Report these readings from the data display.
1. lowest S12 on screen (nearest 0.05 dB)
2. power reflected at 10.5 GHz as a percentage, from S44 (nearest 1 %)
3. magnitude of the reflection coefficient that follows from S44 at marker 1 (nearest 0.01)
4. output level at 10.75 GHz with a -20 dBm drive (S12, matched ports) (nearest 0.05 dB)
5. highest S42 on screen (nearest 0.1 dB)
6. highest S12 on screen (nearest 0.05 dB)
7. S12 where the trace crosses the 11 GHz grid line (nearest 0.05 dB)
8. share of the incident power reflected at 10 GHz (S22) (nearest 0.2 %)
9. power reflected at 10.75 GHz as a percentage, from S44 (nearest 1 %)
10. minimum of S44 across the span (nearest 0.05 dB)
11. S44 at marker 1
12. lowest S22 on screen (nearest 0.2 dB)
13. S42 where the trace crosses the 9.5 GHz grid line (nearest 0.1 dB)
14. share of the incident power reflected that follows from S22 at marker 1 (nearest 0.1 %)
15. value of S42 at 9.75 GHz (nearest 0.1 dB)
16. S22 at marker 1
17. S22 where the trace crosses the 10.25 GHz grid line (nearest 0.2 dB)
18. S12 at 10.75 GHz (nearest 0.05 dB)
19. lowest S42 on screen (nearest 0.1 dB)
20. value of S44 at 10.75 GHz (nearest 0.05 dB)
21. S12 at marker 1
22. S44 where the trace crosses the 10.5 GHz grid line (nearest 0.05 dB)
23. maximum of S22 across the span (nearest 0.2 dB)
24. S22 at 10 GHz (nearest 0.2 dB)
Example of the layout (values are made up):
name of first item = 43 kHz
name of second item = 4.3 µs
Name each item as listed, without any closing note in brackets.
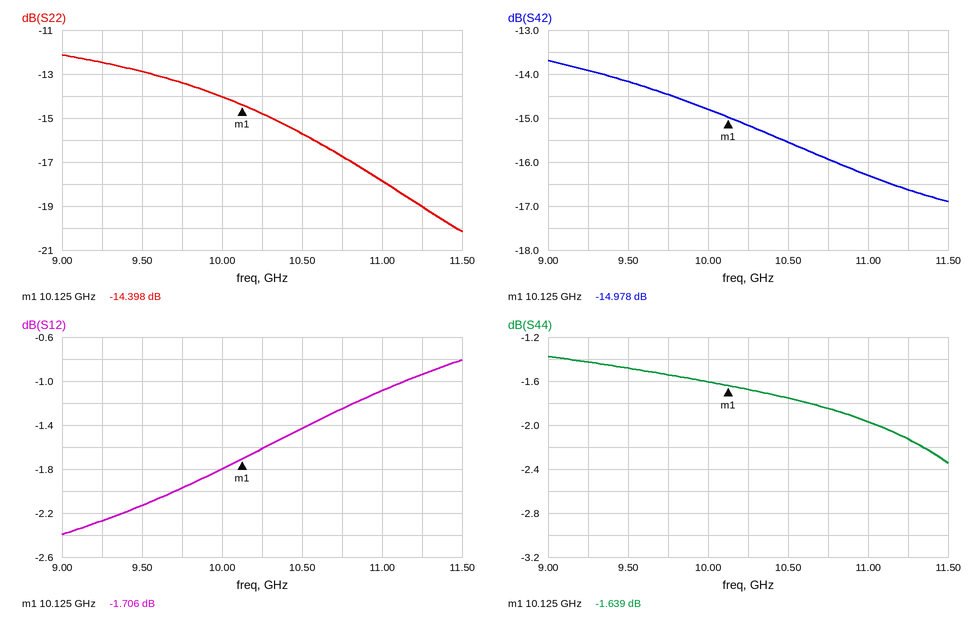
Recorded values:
lowest S12 on screen = -2.40 dB
power reflected at 10.5 GHz as a percentage, from S44 = 67 %
magnitude of the reflection coefficient that follows from S44 at marker 1 = 0.83
output level at 10.75 GHz with a -20 dBm drive (S12, matched ports) = -21.25 dBm
highest S42 on screen = -13.7 dB
highest S12 on screen = -0.80 dB
S12 where the trace crosses the 11 GHz grid line = -1.10 dB
share of the incident power reflected at 10 GHz (S22) = 4.0 %
power reflected at 10.75 GHz as a percentage, from S44 = 65 %
minimum of S44 across the span = -2.35 dB
S44 at marker 1 = -1.639 dB
lowest S22 on screen = -20.2 dB
S42 where the trace crosses the 9.5 GHz grid line = -14.2 dB
share of the incident power reflected that follows from S22 at marker 1 = 3.6 %
value of S42 at 9.75 GHz = -14.5 dB
S22 at marker 1 = -14.398 dB
S22 where the trace crosses the 10.25 GHz grid line = -14.8 dB
S12 at 10.75 GHz = -1.25 dB
lowest S42 on screen = -16.9 dB
value of S44 at 10.75 GHz = -1.85 dB
S12 at marker 1 = -1.706 dB
S44 where the trace crosses the 10.5 GHz grid line = -1.75 dB
maximum of S22 across the span = -12.2 dB
S22 at 10 GHz = -14.0 dB
